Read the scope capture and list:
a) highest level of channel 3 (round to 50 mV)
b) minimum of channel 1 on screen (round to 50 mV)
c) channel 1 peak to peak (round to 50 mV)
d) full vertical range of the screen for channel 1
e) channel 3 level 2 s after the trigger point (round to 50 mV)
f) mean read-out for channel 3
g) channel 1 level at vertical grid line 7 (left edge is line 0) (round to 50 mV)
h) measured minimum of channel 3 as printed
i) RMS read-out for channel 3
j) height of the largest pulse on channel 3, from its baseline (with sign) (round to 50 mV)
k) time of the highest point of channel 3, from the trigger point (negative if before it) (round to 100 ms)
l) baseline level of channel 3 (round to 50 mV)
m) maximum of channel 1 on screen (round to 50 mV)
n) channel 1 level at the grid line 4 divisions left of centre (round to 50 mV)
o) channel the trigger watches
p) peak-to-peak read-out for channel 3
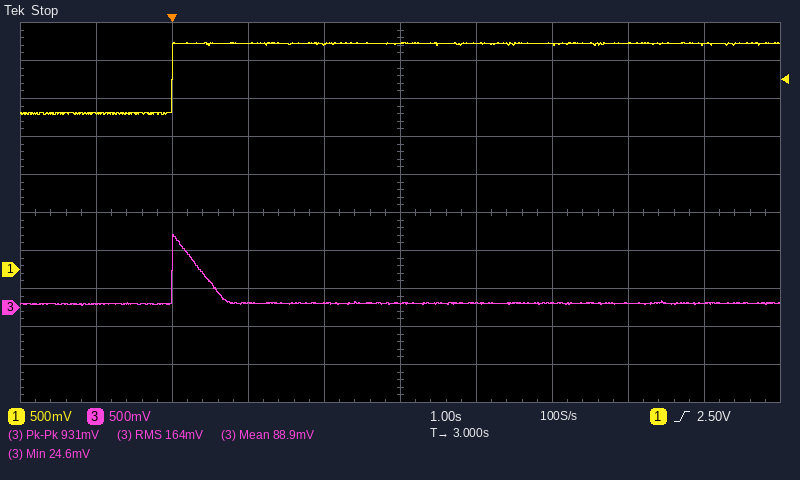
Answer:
950 mV
2.05 V
950 mV
5 V
50 mV
88.9 mV
2.95 V
24.6 mV
164 mV
+900 mV
0.0 s
50 mV
3.00 V
2.05 V
channel 1
931 mV
